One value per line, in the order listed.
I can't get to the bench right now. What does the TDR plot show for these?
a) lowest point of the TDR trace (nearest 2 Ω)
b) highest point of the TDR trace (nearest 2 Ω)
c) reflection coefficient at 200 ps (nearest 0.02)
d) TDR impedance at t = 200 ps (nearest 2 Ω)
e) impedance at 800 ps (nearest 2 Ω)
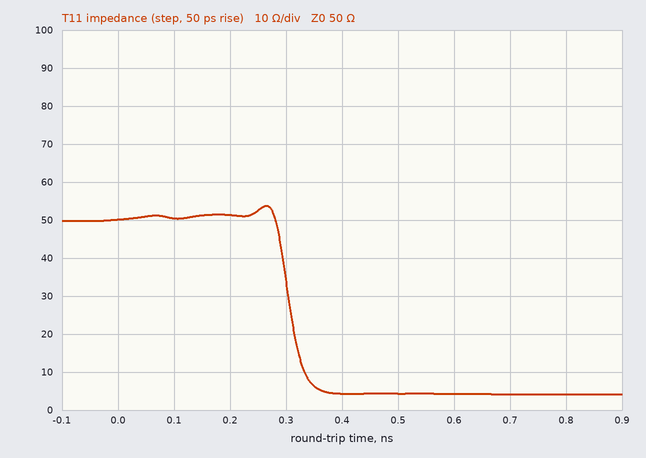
4 Ω
54 Ω
+0.02
52 Ω
4 Ω
